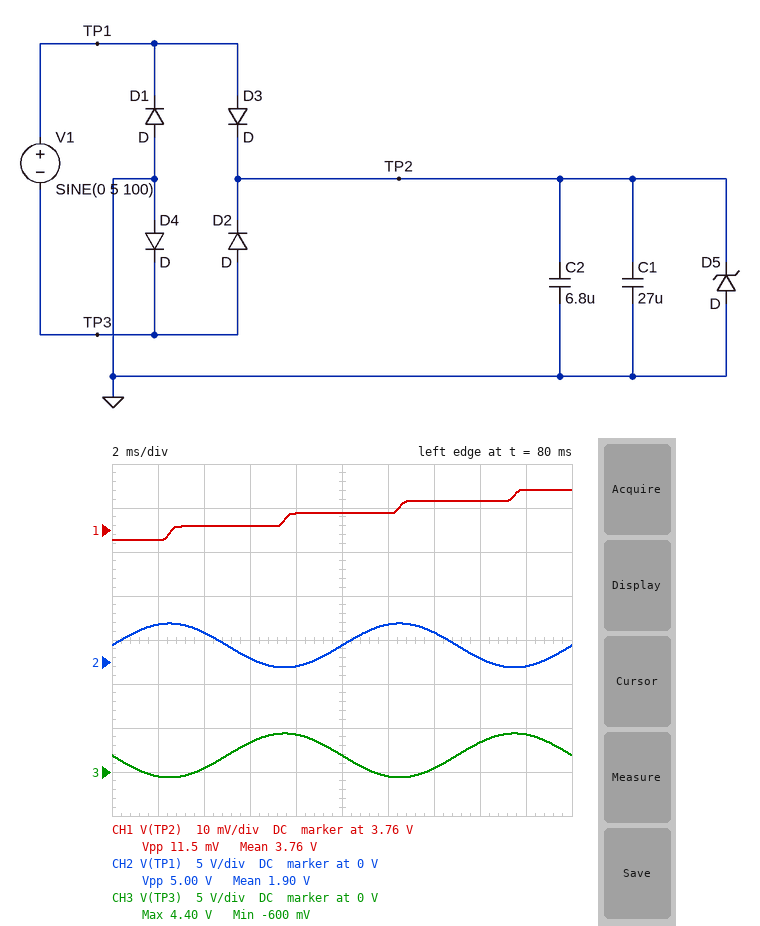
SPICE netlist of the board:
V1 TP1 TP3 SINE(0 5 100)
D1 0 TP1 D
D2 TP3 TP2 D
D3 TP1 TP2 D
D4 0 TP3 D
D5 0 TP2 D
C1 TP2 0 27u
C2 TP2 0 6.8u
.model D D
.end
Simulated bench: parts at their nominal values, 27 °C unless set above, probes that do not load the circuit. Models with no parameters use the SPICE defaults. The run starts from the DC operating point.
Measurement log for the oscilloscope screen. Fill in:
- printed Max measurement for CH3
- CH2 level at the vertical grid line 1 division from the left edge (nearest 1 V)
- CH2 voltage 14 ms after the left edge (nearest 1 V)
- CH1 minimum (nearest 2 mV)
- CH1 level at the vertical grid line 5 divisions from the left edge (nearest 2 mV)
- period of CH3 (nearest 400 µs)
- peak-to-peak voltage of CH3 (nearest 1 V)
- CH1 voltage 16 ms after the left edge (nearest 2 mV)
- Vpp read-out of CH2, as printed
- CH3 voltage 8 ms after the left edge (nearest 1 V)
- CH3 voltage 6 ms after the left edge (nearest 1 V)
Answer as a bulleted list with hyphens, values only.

- 4.40 V
- 4 V
- 3 V
- 3.758 V
- 3.764 V
- 10.0 ms
- 5 V
- 3.766 V
- 5.00 V
- 4 V
- 3 V
